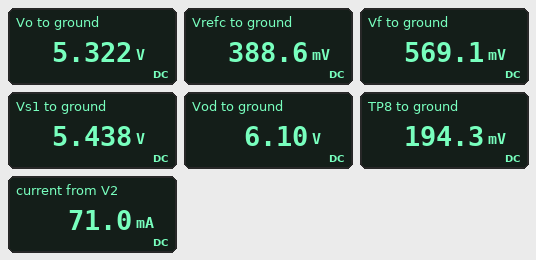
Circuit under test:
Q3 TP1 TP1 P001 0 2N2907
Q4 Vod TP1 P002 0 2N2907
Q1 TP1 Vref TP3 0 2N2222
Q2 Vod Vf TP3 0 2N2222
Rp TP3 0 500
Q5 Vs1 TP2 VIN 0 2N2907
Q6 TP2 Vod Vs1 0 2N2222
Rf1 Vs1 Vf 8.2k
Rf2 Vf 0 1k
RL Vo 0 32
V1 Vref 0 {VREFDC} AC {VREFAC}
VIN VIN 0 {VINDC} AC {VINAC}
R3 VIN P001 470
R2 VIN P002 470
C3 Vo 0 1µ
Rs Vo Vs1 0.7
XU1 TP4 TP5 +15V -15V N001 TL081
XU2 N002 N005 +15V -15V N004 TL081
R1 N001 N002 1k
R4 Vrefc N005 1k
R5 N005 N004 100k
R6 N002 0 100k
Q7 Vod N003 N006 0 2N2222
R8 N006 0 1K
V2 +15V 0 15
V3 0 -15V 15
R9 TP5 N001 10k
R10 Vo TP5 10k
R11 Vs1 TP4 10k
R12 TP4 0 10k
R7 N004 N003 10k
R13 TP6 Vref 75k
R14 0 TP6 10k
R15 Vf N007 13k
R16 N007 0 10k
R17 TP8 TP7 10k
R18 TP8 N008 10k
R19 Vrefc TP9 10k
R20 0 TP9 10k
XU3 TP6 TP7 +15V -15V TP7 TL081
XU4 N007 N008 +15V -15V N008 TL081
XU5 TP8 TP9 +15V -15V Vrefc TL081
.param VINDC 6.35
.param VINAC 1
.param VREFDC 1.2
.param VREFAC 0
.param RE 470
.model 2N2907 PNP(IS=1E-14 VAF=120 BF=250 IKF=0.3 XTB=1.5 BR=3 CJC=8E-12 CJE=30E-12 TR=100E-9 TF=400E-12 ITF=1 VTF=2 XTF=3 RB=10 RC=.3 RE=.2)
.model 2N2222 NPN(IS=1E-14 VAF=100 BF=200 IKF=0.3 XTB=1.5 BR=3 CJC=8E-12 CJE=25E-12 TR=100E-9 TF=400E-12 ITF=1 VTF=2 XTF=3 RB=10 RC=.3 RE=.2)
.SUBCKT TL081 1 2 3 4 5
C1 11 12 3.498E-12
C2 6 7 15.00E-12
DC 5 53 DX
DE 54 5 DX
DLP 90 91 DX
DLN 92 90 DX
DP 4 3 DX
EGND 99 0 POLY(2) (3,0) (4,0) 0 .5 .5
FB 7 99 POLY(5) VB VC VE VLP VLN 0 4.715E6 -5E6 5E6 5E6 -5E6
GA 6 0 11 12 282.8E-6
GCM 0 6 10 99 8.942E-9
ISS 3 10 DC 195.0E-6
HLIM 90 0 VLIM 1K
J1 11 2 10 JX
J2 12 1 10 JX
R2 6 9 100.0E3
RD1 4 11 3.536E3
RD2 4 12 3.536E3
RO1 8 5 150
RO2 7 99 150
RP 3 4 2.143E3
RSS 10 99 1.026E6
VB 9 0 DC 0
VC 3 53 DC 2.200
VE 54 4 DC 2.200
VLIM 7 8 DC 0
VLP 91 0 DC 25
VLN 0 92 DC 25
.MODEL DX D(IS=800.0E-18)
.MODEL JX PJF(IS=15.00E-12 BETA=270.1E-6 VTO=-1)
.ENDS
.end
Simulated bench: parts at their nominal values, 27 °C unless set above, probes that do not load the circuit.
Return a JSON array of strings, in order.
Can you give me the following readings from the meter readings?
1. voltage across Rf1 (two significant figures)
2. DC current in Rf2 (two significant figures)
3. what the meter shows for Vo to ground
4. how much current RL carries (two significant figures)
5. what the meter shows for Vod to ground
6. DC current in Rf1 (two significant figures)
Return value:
["4.9 V", "570 µA", "5.322 V", "170 mA", "6.10 V", "590 µA"]
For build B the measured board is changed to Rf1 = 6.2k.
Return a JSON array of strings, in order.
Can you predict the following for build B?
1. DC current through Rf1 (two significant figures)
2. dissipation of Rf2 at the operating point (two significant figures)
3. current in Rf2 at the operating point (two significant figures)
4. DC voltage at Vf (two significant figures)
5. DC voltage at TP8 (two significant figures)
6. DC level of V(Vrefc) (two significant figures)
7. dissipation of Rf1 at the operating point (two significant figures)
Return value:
["760 µA", "530 µW", "730 µA", "730 mV", "230 mV", "460 mV", "3.6 mW"]
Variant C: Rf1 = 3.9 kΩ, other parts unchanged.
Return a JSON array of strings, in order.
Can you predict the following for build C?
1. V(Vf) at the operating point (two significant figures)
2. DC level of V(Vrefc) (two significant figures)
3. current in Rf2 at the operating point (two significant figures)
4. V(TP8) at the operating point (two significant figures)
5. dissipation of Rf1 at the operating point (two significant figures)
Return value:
["1.1 V", "610 mV", "1.1 mA", "300 mV", "4.9 mW"]
